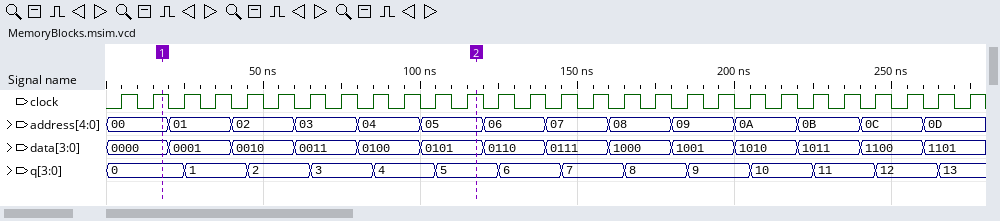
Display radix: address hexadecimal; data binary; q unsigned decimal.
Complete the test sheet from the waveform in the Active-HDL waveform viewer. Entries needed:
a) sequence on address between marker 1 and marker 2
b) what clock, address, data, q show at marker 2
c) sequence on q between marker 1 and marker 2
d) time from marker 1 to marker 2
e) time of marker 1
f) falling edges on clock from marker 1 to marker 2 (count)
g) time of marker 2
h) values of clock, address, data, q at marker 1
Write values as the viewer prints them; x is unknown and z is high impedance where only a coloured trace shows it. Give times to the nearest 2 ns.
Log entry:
00, 01, 02, 03, 04, 05
clock=1, address=05, data=0101, q=5
0, 1, 2, 3, 4, 5
100 ns
18 ns
10
118 ns
clock=1, address=00, data=0000, q=0
